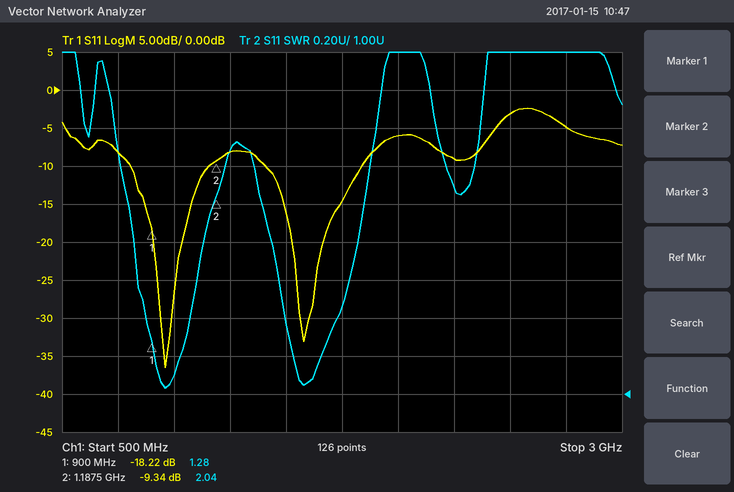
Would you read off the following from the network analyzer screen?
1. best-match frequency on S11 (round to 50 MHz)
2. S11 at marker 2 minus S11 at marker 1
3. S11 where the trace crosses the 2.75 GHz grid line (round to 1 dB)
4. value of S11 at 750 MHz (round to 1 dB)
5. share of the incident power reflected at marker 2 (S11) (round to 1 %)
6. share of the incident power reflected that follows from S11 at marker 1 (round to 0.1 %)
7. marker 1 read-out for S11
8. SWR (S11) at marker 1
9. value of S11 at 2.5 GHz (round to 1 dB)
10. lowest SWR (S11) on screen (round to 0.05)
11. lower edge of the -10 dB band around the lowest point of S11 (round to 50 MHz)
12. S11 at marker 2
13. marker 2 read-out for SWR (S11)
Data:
950 MHz
8.88 dB
-5 dB
-8 dB
12 %
1.5 %
-18.22 dB
1.28
-3 dB
1.05
800 MHz
-9.34 dB
2.04
